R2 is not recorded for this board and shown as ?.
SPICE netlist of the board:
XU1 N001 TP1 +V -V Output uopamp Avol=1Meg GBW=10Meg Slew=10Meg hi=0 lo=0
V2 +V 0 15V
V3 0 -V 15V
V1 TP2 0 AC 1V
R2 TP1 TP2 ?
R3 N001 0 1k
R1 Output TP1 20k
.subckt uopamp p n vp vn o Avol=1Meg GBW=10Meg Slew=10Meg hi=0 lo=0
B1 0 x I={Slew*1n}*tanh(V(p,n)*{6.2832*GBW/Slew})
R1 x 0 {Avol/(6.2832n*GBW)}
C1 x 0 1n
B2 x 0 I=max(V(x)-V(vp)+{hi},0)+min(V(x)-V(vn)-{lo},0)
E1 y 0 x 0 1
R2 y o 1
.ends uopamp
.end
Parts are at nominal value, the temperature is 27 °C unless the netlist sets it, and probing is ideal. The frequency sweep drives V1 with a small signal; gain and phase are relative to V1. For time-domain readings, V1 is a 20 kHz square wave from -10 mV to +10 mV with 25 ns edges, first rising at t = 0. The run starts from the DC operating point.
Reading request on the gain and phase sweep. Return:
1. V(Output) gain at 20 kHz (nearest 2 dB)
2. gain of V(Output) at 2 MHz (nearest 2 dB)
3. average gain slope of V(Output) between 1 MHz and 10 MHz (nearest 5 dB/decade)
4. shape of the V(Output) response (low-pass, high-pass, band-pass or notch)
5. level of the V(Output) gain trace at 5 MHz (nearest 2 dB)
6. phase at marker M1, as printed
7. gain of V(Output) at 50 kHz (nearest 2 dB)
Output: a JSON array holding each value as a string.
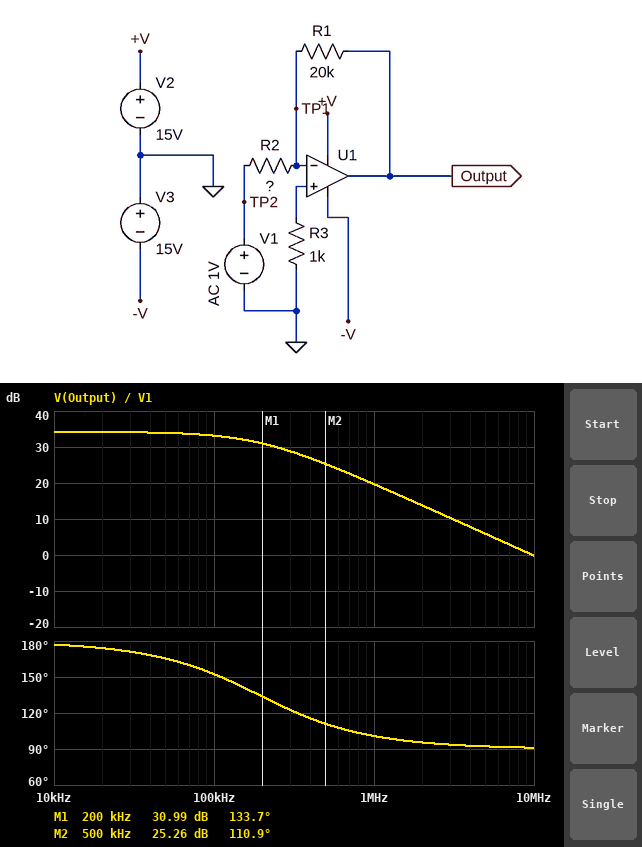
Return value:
["34 dB", "14 dB", "-20 dB/decade", "low-pass", "6 dB", "133.7 deg", "34 dB"]
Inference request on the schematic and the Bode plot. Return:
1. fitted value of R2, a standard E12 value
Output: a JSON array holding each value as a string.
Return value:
["390 Ω"]
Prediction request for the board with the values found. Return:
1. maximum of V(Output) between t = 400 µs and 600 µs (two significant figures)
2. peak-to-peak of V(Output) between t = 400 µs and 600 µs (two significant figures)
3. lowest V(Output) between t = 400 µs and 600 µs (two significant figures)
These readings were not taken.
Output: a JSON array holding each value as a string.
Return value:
["510 mV", "1.0 V", "-510 mV"]
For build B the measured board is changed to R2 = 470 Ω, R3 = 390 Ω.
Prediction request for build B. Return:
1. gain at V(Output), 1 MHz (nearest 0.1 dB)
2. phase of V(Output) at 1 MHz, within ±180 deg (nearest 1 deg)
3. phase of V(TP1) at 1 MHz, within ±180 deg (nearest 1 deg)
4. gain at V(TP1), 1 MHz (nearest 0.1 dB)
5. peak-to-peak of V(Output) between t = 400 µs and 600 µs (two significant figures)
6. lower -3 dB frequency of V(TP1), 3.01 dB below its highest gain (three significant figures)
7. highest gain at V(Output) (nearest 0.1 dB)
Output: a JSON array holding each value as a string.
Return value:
["19.6 dB", "103 deg", "13 deg", "-0.4 dB", "850 mV", "230 kHz", "32.6 dB"]
